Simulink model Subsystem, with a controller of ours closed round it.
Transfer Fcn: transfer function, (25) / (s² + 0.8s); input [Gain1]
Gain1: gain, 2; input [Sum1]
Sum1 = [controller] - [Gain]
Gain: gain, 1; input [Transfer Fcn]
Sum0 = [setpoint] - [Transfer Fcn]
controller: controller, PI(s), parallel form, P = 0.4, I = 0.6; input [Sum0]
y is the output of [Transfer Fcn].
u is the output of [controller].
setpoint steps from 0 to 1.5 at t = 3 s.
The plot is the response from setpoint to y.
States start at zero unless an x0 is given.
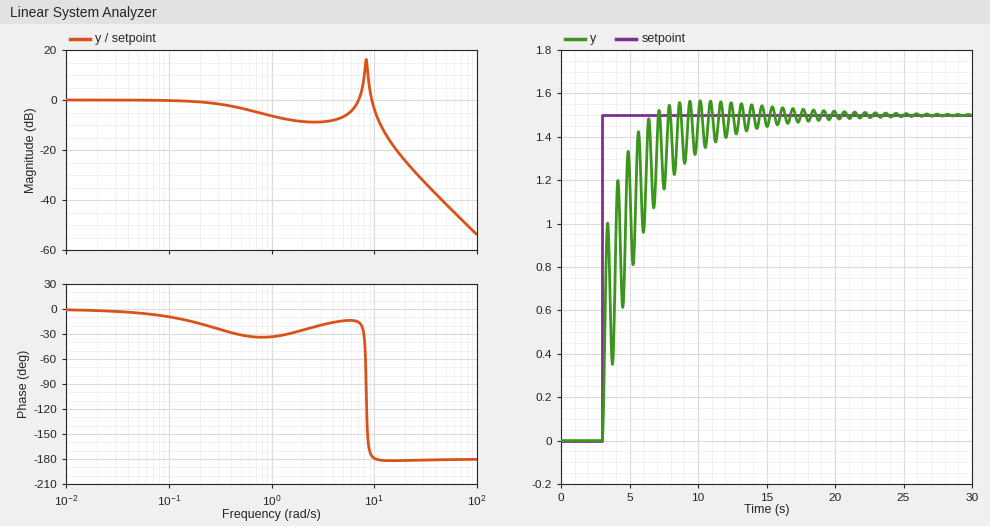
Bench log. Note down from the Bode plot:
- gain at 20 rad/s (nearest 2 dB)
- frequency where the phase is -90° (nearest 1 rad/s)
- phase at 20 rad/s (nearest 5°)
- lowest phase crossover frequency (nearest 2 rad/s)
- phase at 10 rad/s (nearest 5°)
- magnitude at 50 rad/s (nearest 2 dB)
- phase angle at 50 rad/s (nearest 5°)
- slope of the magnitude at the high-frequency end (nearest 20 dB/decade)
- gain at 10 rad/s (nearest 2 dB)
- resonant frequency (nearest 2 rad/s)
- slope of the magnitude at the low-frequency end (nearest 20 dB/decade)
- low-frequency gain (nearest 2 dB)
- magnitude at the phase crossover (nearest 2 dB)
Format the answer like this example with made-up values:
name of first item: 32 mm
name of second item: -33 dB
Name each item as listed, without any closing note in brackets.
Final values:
gain at 20 rad/s: -24 dB
frequency where the phase is -90°: 8 rad/s
phase at 20 rad/s: -180°
lowest phase crossover frequency: 10 rad/s
phase at 10 rad/s: -180°
magnitude at 50 rad/s: -42 dB
phase angle at 50 rad/s: -180°
slope of the magnitude at the high-frequency end: -40 dB/decade
gain at 10 rad/s: -4 dB
resonant frequency: 8 rad/s
slope of the magnitude at the low-frequency end: 0 dB/decade
low-frequency gain: 0 dB
magnitude at the phase crossover: -6 dB
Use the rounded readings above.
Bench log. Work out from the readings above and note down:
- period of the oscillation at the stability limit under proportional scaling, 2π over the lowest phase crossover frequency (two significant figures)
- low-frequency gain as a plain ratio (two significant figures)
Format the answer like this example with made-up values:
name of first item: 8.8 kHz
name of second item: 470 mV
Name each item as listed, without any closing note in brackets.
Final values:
period of the oscillation at the stability limit under proportional scaling, 2π over the lowest phase crossover frequency: 0.63 s
low-frequency gain as a plain ratio: 1.0
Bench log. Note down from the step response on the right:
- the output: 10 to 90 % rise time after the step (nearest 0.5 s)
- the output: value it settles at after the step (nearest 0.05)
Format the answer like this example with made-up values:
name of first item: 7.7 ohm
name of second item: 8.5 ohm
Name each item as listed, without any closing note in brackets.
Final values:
the output: 10 to 90 % rise time after the step: 2.5 s
the output: value it settles at after the step: 1.50
